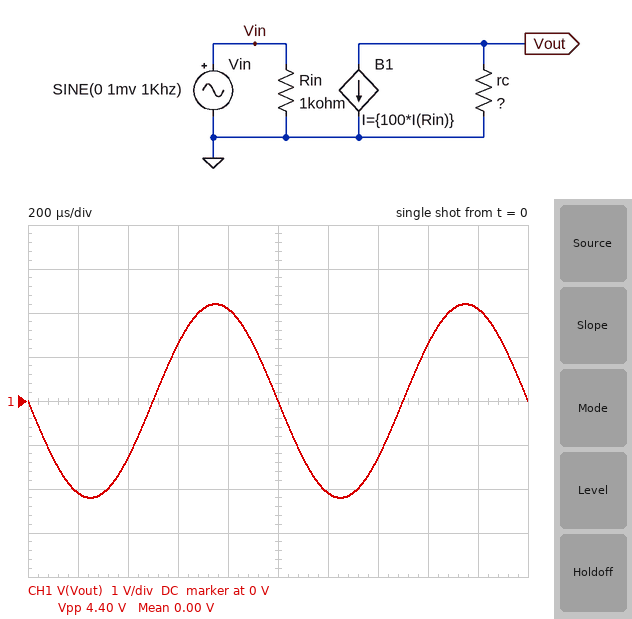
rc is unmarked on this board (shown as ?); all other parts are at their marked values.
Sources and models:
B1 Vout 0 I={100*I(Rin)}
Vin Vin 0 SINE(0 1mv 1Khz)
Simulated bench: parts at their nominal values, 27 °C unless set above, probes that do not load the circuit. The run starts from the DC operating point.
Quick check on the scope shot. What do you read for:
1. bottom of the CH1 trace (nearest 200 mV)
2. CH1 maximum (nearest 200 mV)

-2.2 V
2.2 V
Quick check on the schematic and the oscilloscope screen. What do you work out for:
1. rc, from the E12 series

22 kΩ
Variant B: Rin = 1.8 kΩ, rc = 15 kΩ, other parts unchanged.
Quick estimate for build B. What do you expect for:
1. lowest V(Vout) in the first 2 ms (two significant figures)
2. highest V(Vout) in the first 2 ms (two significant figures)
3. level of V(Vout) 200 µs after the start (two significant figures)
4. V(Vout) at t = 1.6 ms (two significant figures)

-830 mV
830 mV
-790 mV
490 mV
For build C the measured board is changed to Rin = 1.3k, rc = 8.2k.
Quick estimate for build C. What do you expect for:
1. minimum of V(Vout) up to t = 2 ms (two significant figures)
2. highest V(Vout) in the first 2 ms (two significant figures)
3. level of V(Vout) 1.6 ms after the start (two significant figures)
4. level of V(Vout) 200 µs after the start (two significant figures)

-630 mV
630 mV
370 mV
-600 mV
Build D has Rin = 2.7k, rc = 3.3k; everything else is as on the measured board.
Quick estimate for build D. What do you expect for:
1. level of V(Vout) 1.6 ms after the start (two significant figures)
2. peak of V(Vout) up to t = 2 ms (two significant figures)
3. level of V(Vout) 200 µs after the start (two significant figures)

72 mV
120 mV
-120 mV
